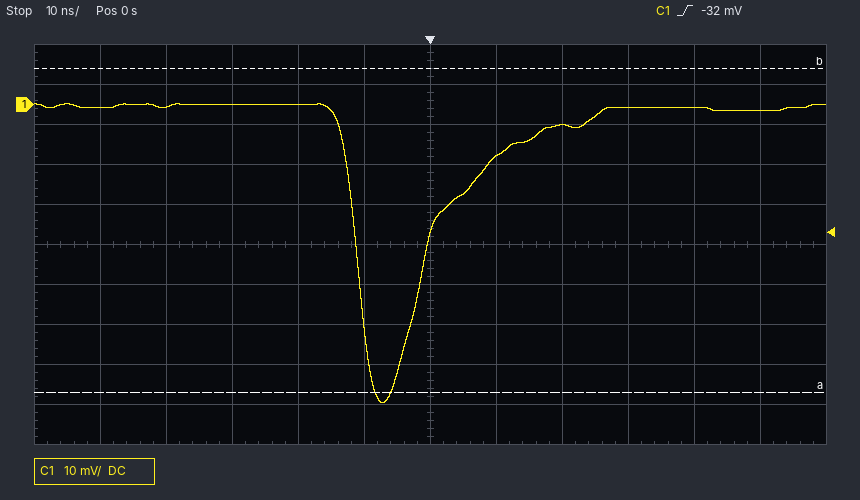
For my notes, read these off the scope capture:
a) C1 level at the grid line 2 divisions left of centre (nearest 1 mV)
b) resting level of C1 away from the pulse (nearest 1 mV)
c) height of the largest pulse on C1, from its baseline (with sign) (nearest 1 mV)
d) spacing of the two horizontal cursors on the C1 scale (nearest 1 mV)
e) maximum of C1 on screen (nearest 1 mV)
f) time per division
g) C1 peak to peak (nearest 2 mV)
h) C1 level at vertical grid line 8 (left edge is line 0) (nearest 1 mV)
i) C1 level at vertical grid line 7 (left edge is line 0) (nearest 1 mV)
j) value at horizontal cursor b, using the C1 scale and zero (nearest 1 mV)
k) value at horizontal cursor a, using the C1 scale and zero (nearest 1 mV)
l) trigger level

0 mV
-1 mV
-74 mV
81 mV
0 mV
10 ns
74 mV
-5 mV
-13 mV
9 mV
-72 mV
-32 mV
